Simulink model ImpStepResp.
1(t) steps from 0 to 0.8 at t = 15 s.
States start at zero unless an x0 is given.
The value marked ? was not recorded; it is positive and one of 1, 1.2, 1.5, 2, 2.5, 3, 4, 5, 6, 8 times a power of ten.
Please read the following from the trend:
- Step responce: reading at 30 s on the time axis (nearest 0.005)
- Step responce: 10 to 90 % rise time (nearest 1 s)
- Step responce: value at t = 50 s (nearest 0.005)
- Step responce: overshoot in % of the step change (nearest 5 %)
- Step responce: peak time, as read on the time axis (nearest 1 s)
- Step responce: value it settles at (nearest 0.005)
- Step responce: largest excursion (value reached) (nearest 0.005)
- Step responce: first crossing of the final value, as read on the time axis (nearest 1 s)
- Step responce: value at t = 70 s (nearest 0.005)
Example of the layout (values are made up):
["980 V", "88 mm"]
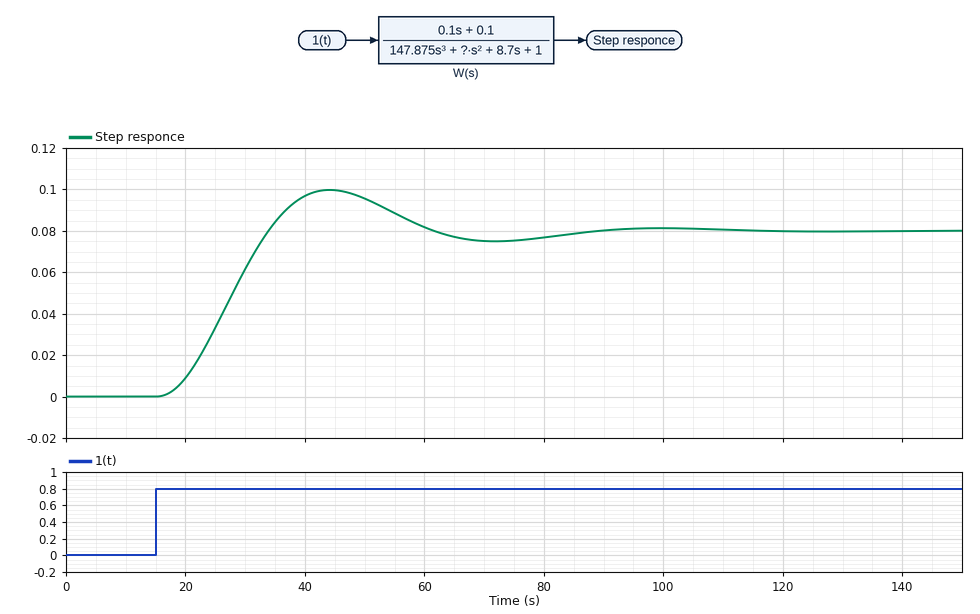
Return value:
["0.060", "12 s", "0.095", "25 %", "44 s", "0.080", "0.100", "34 s", "0.075"]
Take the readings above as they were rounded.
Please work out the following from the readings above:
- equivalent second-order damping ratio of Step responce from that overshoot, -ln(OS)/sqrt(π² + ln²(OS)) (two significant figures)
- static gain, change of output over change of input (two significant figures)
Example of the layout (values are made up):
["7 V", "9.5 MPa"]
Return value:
["0.40", "0.10"]
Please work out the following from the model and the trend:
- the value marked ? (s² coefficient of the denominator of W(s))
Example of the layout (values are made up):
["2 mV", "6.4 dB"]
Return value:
["80"]
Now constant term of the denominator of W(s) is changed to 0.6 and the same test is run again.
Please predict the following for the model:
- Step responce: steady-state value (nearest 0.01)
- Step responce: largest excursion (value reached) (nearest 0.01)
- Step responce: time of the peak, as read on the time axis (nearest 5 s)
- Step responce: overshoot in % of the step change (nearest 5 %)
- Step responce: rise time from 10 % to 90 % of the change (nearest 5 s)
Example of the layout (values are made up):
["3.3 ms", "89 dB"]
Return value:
["0.13", "0.15", "55 s", "10 %", "20 s"]
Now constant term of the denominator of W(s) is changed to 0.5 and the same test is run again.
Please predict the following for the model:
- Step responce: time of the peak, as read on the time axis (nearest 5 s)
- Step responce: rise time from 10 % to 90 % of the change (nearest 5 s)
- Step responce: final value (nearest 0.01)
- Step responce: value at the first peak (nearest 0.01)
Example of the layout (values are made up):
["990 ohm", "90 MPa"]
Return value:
["65 s", "25 s", "0.16", "0.17"]
